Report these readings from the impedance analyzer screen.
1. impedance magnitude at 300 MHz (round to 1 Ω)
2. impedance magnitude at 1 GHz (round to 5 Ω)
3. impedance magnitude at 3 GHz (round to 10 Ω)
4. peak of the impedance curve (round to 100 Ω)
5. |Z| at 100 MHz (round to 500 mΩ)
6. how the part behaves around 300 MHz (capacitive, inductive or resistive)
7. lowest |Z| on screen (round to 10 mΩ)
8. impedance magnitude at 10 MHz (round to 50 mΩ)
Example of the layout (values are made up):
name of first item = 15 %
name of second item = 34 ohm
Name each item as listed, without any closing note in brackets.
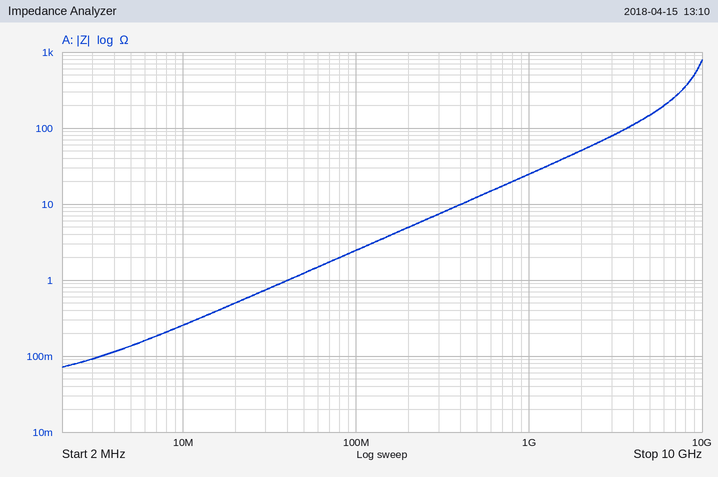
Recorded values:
impedance magnitude at 300 MHz = 7 Ω
impedance magnitude at 1 GHz = 25 Ω
impedance magnitude at 3 GHz = 80 Ω
peak of the impedance curve = 800 Ω
|Z| at 100 MHz = 2.5 Ω
how the part behaves around 300 MHz = inductive
lowest |Z| on screen = 70 mΩ
impedance magnitude at 10 MHz = 250 mΩ
